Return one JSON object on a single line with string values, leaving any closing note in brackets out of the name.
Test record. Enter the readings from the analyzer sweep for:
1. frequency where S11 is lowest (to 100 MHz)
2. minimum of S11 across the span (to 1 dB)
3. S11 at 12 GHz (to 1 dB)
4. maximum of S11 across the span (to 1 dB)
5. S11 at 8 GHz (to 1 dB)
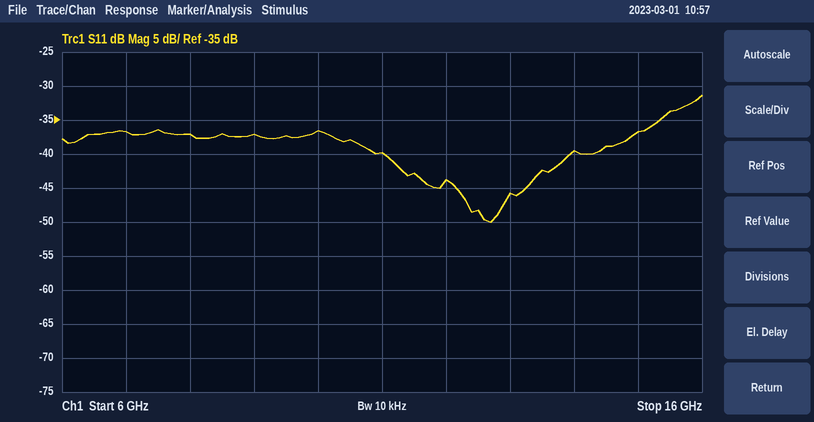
{"frequency where S11 is lowest": "12.7 GHz", "minimum of S11 across the span": "-50 dB", "S11 at 12 GHz": "-44 dB", "maximum of S11 across the span": "-31 dB", "S11 at 8 GHz": "-37 dB"}
